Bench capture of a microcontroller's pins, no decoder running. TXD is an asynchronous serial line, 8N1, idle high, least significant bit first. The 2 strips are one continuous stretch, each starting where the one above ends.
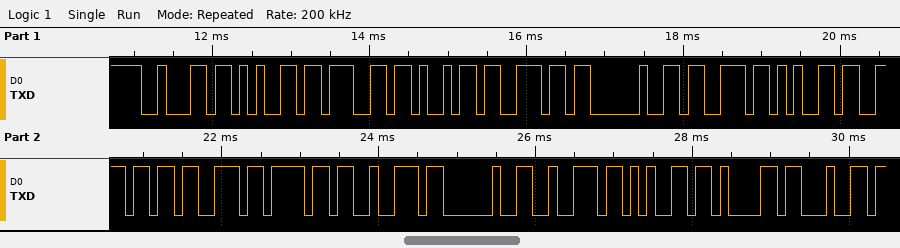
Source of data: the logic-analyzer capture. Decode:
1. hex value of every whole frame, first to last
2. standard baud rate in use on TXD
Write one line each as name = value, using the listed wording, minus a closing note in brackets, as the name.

hex value of every whole frame, first to last = 0x62 0x65 0x67 0x69 0x6E 0x20 0x73 0x65 0x6E 0x73 0x6F 0x72 0x20 0x72 0x65 0x61 0x64
standard baud rate in use on TXD = 9600 baud
